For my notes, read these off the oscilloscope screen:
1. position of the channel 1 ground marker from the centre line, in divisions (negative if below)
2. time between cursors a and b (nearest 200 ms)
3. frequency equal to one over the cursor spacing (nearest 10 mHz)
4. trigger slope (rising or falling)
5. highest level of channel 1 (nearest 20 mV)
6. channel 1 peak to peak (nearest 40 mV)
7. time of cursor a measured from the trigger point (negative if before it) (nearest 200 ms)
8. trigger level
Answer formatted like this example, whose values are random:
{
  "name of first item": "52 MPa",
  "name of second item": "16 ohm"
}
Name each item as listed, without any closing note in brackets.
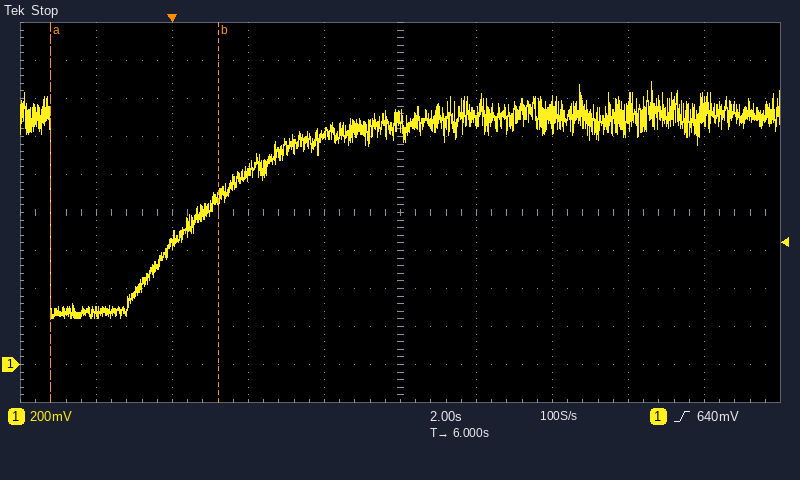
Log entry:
{
  "position of the channel 1 ground marker from the centre line, in divisions": "-4.0 div",
  "time between cursors a and b": "4.4 s",
  "frequency equal to one over the cursor spacing": "230 mHz",
  "trigger slope": "rising",
  "highest level of channel 1": "1.48 V",
  "channel 1 peak to peak": "1.24 V",
  "time of cursor a measured from the trigger point (negative if before it)": "-3.2 s",
  "trigger level": "640 mV"
}
